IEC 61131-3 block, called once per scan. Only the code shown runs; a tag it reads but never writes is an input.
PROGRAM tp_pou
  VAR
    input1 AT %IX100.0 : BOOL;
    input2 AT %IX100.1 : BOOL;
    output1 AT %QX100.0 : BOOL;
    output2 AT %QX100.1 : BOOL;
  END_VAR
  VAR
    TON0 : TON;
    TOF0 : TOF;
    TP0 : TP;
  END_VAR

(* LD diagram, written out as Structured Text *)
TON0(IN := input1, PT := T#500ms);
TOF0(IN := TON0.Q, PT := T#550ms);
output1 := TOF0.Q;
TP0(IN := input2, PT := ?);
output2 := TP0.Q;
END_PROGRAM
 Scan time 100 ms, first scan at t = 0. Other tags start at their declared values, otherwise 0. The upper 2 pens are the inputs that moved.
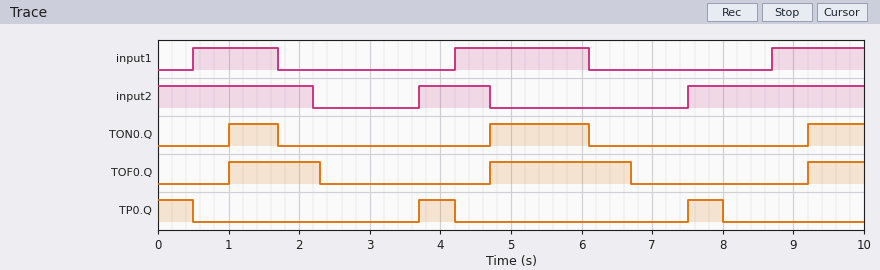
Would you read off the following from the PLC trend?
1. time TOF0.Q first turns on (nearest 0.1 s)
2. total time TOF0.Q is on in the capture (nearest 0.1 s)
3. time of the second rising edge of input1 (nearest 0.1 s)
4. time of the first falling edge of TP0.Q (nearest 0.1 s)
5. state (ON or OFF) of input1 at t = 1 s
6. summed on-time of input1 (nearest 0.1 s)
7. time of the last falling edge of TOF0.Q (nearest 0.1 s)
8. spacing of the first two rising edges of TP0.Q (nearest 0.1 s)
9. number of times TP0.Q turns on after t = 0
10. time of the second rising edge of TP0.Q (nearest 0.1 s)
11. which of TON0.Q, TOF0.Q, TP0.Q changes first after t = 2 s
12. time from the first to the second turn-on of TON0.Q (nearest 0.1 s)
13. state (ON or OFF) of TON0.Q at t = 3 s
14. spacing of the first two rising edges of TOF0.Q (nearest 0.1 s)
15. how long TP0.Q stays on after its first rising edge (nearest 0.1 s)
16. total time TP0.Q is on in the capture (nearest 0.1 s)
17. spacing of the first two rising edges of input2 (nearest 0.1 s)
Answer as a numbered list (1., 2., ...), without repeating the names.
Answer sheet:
1. 1.0 s
2. 4.1 s
3. 4.2 s
4. 0.5 s
5. ON
6. 4.4 s
7. 6.7 s
8. 3.8 s
9. 2
10. 7.5 s
11. TOF0.Q
12. 3.7 s
13. OFF
14. 3.7 s
15. 0.5 s
16. 1.5 s
17. 3.8 s
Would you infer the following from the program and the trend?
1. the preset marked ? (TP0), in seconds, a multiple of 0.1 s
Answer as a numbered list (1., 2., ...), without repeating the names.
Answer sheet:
1. 0.5 s
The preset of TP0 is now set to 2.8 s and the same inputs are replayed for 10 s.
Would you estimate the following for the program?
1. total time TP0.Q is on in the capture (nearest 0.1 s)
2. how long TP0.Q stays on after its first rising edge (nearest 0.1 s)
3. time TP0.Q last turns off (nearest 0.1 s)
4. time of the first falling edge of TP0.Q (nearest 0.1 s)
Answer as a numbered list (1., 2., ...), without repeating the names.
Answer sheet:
1. 8.1 s
2. 2.8 s
3. 6.5 s
4. 2.8 s
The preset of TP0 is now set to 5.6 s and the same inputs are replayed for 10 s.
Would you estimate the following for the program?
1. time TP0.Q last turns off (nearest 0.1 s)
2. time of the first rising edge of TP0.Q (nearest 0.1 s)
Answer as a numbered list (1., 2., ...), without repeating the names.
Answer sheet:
1. 5.6 s
2. 7.5 s
